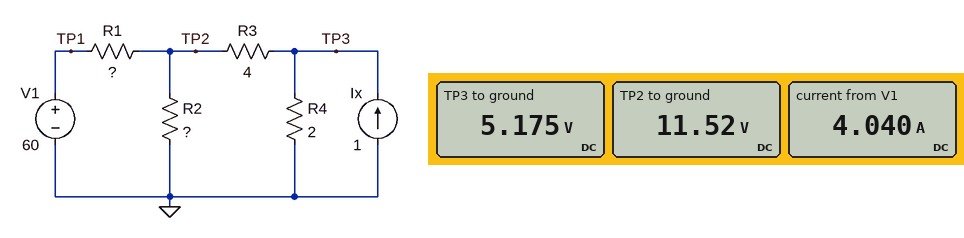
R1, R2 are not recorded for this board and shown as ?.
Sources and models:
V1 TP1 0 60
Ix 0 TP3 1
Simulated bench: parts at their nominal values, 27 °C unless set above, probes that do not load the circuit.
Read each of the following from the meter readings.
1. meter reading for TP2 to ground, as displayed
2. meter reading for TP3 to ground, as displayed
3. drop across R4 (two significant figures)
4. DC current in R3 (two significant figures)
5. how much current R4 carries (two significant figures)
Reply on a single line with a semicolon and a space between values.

11.52 V; 5.175 V; 5.2 V; 1.6 A; 2.6 A
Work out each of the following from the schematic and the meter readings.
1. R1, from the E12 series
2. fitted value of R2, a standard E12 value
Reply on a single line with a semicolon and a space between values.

12 Ω; 4.7 Ω
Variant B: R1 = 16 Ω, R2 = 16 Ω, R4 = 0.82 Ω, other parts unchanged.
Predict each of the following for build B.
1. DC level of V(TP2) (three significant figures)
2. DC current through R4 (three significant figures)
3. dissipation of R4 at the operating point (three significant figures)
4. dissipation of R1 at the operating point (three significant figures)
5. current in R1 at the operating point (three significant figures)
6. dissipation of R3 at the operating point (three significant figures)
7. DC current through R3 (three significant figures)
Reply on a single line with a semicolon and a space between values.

11.8 V; 3.28 A; 8.80 W; 145 W; 3.01 A; 20.7 W; 2.28 A
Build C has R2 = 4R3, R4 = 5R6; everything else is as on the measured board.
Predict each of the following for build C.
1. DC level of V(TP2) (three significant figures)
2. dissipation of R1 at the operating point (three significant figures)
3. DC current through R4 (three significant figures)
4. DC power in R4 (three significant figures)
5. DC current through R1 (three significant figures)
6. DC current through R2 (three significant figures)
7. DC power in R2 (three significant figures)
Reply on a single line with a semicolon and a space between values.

13.3 V; 182 W; 1.80 A; 18.2 W; 3.89 A; 3.09 A; 41.1 W
